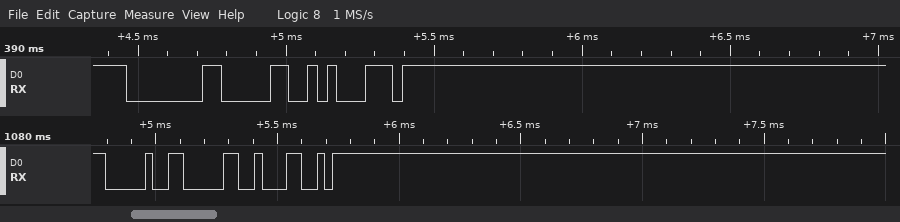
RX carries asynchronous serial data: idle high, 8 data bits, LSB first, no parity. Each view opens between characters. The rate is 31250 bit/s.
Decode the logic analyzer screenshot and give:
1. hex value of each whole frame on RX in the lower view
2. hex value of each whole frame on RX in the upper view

90, 30, 4C
80, 30, 71
